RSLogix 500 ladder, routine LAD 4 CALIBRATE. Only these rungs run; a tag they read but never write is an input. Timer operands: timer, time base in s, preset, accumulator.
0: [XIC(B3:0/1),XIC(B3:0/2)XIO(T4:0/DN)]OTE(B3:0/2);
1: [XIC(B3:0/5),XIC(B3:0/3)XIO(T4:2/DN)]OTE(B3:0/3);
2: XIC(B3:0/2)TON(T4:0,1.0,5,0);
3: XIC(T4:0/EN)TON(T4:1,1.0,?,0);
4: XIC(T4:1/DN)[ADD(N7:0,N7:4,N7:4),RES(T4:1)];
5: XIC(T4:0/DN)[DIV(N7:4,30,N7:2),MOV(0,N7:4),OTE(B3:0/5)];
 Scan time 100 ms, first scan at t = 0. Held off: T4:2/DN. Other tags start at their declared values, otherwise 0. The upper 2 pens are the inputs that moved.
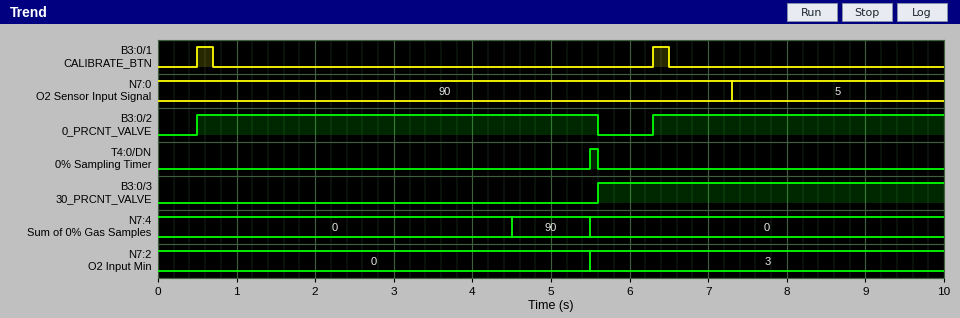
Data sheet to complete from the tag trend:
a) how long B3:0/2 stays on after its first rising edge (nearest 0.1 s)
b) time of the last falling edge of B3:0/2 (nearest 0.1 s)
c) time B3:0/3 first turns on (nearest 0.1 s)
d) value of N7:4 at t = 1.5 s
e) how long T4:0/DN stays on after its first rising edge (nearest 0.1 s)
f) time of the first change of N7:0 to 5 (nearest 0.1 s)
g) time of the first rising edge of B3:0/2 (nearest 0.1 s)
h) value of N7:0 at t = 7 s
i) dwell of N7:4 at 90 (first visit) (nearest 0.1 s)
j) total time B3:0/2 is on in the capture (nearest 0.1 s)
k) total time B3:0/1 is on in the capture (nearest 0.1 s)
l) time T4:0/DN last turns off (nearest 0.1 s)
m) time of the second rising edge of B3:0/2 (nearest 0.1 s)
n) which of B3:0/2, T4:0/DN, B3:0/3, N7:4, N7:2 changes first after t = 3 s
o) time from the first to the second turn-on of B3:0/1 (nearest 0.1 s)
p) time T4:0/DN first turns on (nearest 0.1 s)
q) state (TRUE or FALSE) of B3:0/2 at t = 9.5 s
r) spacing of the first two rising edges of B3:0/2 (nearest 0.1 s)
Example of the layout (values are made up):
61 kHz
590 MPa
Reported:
5.1 s
5.6 s
5.6 s
0
0.1 s
7.3 s
0.5 s
90
1.0 s
8.8 s
0.4 s
5.6 s
6.3 s
N7:4
5.8 s
5.5 s
TRUE
5.8 s
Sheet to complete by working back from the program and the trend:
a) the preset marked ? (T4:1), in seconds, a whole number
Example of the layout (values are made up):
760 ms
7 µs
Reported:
4 s
